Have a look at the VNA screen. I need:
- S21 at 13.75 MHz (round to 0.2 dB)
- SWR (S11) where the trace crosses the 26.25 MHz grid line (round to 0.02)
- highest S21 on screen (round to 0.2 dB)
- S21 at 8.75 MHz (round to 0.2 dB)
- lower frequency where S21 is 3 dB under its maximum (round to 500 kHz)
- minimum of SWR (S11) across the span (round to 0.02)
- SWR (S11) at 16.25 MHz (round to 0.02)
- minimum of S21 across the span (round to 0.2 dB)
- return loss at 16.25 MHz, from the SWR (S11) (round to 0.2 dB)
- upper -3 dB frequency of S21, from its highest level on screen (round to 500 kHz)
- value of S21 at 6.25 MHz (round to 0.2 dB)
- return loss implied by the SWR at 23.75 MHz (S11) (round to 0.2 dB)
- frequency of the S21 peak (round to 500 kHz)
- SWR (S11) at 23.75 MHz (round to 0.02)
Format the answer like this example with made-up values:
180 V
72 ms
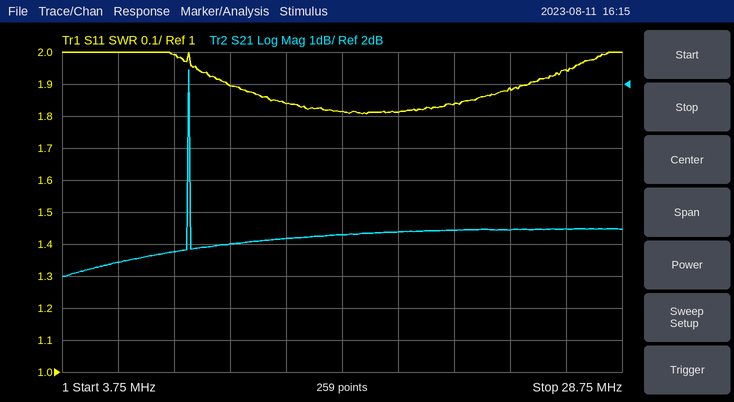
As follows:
-2.8 dB
1.94
2.4 dB
-3.2 dB
9.5 MHz
1.80
1.82
-4.0 dB
10.8 dB
9.5 MHz
-3.6 dB
10.2 dB
9.5 MHz
1.88
